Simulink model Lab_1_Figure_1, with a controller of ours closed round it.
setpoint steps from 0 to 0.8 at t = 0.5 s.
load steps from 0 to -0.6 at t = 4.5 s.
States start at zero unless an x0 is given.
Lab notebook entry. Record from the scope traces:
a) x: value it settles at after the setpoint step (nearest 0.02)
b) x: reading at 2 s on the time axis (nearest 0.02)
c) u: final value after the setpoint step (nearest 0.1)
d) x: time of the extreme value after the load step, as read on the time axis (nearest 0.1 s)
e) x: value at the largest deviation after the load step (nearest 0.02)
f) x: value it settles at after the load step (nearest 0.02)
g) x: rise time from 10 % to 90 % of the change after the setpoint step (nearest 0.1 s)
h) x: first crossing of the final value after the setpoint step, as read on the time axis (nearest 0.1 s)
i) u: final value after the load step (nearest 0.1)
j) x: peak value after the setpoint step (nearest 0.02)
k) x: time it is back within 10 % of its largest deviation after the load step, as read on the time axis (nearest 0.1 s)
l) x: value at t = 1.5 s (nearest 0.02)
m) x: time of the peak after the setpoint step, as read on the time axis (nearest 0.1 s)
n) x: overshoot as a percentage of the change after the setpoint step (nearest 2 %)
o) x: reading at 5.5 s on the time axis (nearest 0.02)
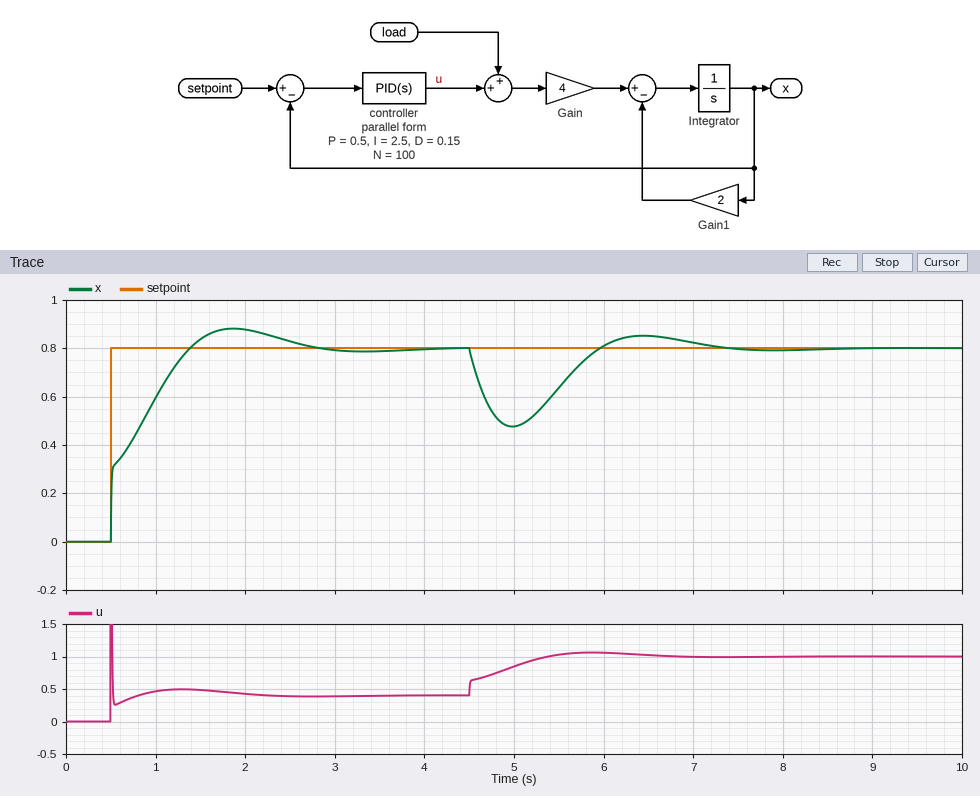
0.80
0.88
0.4
5.0 s
0.48
0.80
0.7 s
1.4 s
1.0
0.88
6.9 s
0.84
1.9 s
10 %
0.64
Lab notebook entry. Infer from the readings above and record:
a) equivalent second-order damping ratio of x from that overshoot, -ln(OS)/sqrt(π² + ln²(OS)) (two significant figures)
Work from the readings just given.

0.59
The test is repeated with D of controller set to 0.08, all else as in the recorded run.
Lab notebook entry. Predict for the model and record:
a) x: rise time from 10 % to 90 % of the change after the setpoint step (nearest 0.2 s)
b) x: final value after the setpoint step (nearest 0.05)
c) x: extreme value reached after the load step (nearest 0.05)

0.6 s
0.80
0.45
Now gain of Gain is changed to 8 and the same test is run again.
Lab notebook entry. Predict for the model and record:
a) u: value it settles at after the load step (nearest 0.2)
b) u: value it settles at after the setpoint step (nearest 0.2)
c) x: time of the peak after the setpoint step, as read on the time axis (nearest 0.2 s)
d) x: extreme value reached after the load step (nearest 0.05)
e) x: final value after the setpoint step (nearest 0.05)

0.8
0.2
1.6 s
0.40
0.80
